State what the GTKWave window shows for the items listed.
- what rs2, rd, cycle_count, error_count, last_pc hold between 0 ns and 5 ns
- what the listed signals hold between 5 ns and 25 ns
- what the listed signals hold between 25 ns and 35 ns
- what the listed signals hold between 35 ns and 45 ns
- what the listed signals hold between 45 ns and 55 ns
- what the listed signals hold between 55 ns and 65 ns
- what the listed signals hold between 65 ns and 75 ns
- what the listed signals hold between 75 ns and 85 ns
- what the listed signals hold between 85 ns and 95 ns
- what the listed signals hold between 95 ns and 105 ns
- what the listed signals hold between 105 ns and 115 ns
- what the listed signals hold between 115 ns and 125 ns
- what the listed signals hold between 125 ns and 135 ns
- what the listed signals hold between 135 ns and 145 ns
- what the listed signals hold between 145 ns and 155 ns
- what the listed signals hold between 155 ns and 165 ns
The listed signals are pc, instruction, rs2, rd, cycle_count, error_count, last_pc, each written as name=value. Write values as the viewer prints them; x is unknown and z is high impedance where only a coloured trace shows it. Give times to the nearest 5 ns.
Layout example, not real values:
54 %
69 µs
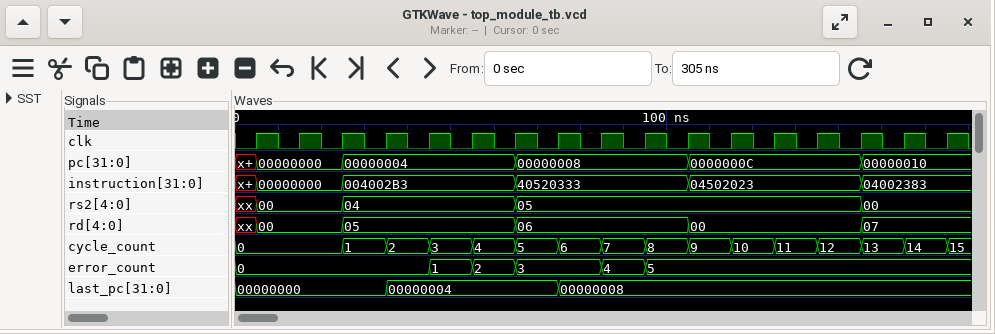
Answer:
rs2=xx, rd=xx, cycle_count=0, error_count=0, last_pc=00000000
pc=00000000, instruction=00000000, rs2=00, rd=00, cycle_count=0, error_count=0, last_pc=00000000
pc=00000004, instruction=004002B3, rs2=04, rd=05, cycle_count=1, error_count=0, last_pc=00000000
pc=00000004, instruction=004002B3, rs2=04, rd=05, cycle_count=2, error_count=0, last_pc=00000004
pc=00000004, instruction=004002B3, rs2=04, rd=05, cycle_count=3, error_count=1, last_pc=00000004
pc=00000004, instruction=004002B3, rs2=04, rd=05, cycle_count=4, error_count=2, last_pc=00000004
pc=00000008, instruction=40520333, rs2=05, rd=06, cycle_count=5, error_count=3, last_pc=00000004
pc=00000008, instruction=40520333, rs2=05, rd=06, cycle_count=6, error_count=3, last_pc=00000008
pc=00000008, instruction=40520333, rs2=05, rd=06, cycle_count=7, error_count=4, last_pc=00000008
pc=00000008, instruction=40520333, rs2=05, rd=06, cycle_count=8, error_count=5, last_pc=00000008
pc=0000000C, instruction=04502023, rs2=05, rd=00, cycle_count=9, error_count=5, last_pc=00000008
pc=0000000C, instruction=04502023, rs2=05, rd=00, cycle_count=10, error_count=5, last_pc=00000008
pc=0000000C, instruction=04502023, rs2=05, rd=00, cycle_count=11, error_count=5, last_pc=00000008
pc=0000000C, instruction=04502023, rs2=05, rd=00, cycle_count=12, error_count=5, last_pc=00000008
pc=00000010, instruction=04002383, rs2=00, rd=07, cycle_count=13, error_count=5, last_pc=00000008
pc=00000010, instruction=04002383, rs2=00, rd=07, cycle_count=14, error_count=5, last_pc=00000008
